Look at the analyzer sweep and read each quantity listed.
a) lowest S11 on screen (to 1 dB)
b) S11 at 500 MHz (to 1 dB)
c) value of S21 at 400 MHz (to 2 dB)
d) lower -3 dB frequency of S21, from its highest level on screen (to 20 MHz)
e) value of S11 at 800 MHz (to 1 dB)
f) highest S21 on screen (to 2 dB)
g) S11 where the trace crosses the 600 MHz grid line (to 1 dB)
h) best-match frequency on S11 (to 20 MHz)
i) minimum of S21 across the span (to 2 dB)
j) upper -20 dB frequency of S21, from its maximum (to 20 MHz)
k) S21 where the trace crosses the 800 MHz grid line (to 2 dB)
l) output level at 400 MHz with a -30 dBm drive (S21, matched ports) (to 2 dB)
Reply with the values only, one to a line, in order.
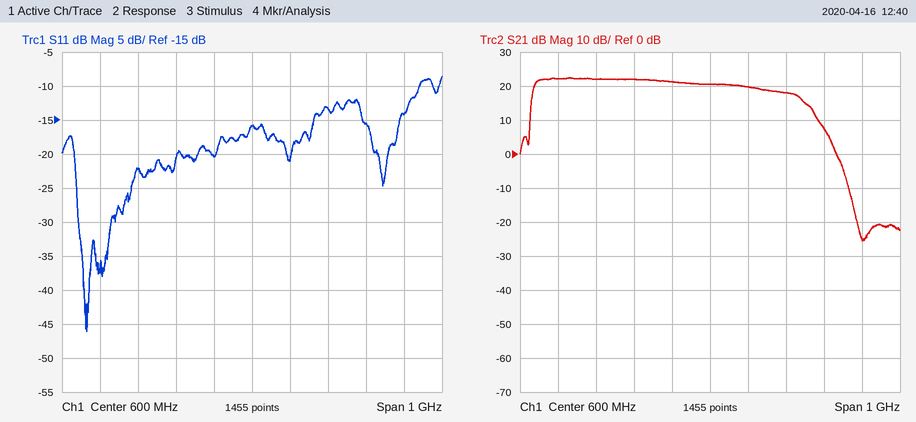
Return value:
-46 dB
-20 dB
22 dB
140 MHz
-13 dB
22 dB
-16 dB
160 MHz
-26 dB
920 MHz
18 dB
-8 dBm
